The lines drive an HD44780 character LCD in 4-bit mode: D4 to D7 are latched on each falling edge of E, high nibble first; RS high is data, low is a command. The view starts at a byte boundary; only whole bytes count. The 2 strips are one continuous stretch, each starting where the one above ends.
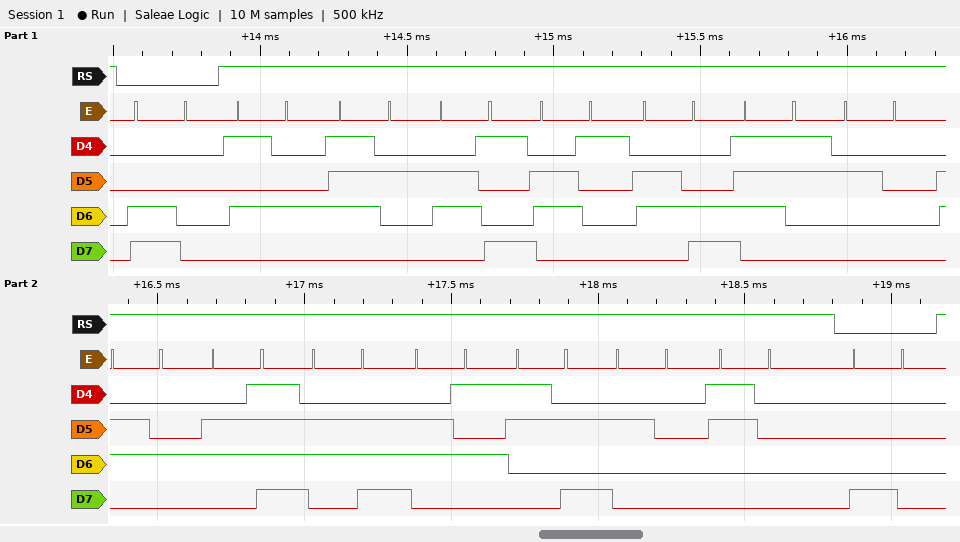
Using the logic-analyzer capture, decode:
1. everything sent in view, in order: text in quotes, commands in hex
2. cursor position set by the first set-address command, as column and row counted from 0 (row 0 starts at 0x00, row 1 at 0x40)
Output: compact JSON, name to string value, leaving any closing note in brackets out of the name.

{"everything sent in view, in order: text in quotes, commands in hex": "0xC0 \"Trials done: 0\" 0x80", "cursor position set by the first set-address command, as column and row counted from 0": "column 0, row 1"}
